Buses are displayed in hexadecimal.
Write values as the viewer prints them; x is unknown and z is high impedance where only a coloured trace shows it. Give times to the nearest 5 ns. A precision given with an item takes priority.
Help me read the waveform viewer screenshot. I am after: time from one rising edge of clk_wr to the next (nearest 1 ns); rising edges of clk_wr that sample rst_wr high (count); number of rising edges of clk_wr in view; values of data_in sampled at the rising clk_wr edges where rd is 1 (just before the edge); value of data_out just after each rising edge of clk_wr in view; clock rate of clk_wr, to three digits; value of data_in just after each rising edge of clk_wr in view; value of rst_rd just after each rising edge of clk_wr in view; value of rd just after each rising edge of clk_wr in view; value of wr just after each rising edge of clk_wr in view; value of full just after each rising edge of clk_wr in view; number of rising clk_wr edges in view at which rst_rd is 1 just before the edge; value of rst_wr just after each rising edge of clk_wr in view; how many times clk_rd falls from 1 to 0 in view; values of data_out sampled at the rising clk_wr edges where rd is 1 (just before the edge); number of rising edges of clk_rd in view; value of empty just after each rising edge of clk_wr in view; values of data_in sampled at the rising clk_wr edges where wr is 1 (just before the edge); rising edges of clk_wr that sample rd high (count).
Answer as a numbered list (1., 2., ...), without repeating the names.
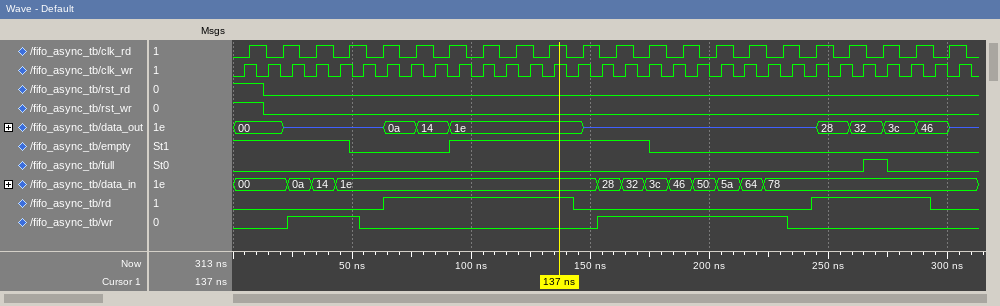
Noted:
1. 10 ns
2. 1
3. 31
4. 1e, 1e, 1e, 1e, 1e, 1e, 1e, 1e, 78, 78, 78, 78, 78
5. 00, 00, z, z, z, z, 0a, 0a, 14, 1e, 1e, 1e, 1e, 1e, 1e, z, z, z, z, z, z, z, z, z, 28, 28, 32, 3c, 3c, 46, z
6. 100 MHz
7. 00, 00, 0a, 14, 1e, 1e, 1e, 1e, 1e, 1e, 1e, 1e, 1e, 1e, 1e, 28, 32, 3c, 46, 50, 5a, 64, 78, 78, 78, 78, 78, 78, 78, 78, 78
8. 1 0 0 0 0 0 0 0 0 0 0 0 0 0 0 0 0 0 0 0 0 0 0 0 0 0 0 0 0 0 0
9. 0 0 0 0 0 0 1 1 1 1 1 1 1 1 0 0 0 0 0 0 0 0 0 0 1 1 1 1 1 0 0
10. 0 0 1 1 1 0 0 0 0 0 0 0 0 0 0 1 1 1 1 1 1 1 1 0 0 0 0 0 0 0 0
11. 0 0 0 0 0 0 0 0 0 0 0 0 0 0 0 0 0 0 0 0 0 0 0 0 0 0 1 0 0 0 0
12. 1
13. 1 0 0 0 0 0 0 0 0 0 0 0 0 0 0 0 0 0 0 0 0 0 0 0 0 0 0 0 0 0 0
14. 22
15. 0a, 0a, 14, 1e, 1e, 1e, 1e, 1e, z, 28, 32, 3c, 3c
16. 22
17. 1 1 1 1 1 0 0 0 0 1 1 1 1 1 1 1 1 0 0 0 0 0 0 0 0 0 0 0 0 0 0
18. 0a, 14, 1e, 28, 32, 3c, 46, 50, 5a, 64, 78
19. 13
